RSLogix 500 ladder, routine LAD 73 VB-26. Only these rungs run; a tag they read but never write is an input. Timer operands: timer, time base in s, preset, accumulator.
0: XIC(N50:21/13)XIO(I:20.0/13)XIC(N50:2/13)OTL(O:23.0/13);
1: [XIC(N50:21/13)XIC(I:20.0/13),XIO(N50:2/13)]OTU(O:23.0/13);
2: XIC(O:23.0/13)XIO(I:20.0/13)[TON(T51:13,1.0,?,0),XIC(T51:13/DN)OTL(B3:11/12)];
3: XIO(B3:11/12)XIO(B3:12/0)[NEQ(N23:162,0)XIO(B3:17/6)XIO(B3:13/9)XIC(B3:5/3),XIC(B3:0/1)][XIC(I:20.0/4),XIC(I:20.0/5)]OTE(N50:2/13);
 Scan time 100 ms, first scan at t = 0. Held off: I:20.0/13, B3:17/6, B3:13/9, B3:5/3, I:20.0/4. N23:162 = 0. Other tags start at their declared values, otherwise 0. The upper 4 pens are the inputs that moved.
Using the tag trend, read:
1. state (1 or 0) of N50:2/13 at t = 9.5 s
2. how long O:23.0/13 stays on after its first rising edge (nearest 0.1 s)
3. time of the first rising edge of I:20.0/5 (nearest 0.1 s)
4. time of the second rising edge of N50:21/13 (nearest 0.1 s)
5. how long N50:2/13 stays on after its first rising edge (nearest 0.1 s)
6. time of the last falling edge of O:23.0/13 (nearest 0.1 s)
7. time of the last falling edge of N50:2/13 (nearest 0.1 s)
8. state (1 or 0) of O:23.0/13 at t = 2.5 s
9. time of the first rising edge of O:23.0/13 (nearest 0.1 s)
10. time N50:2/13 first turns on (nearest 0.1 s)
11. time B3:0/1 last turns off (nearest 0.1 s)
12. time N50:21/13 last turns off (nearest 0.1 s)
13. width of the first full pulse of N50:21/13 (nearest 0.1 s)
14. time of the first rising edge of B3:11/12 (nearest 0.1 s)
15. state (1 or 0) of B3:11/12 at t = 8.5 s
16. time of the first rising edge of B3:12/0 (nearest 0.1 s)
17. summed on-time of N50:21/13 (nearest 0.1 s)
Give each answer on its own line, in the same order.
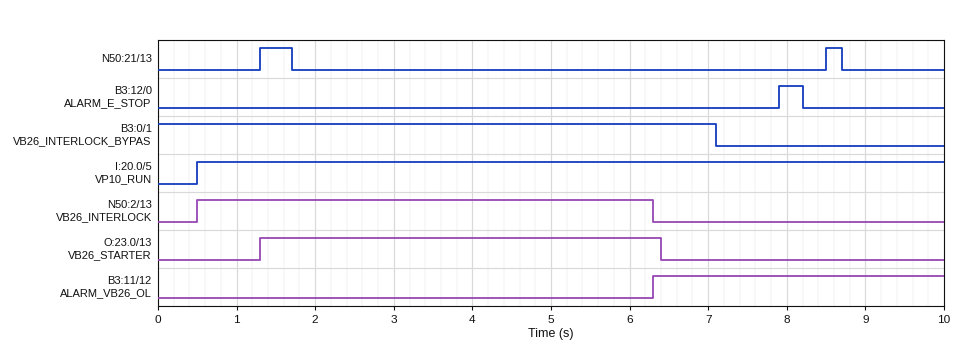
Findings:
0
5.1 s
0.5 s
8.5 s
5.8 s
6.4 s
6.3 s
1
1.3 s
0.5 s
7.1 s
8.7 s
0.4 s
6.3 s
1
7.9 s
0.6 s
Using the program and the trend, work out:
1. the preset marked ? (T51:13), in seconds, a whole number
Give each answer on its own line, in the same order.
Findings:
5 s
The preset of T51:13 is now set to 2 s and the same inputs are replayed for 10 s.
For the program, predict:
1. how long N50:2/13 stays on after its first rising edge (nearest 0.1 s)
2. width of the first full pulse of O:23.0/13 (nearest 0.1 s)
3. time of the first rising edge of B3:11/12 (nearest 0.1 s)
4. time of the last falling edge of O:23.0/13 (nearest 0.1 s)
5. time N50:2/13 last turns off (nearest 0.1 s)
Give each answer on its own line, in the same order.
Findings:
2.8 s
2.1 s
3.3 s
3.4 s
3.3 s
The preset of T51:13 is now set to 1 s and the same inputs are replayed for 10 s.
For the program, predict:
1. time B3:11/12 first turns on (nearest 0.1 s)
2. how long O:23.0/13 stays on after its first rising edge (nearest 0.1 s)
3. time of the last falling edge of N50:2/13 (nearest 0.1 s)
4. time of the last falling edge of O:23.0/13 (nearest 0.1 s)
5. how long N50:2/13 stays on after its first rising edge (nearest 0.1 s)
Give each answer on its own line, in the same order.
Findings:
2.3 s
1.1 s
2.3 s
2.4 s
1.8 s
